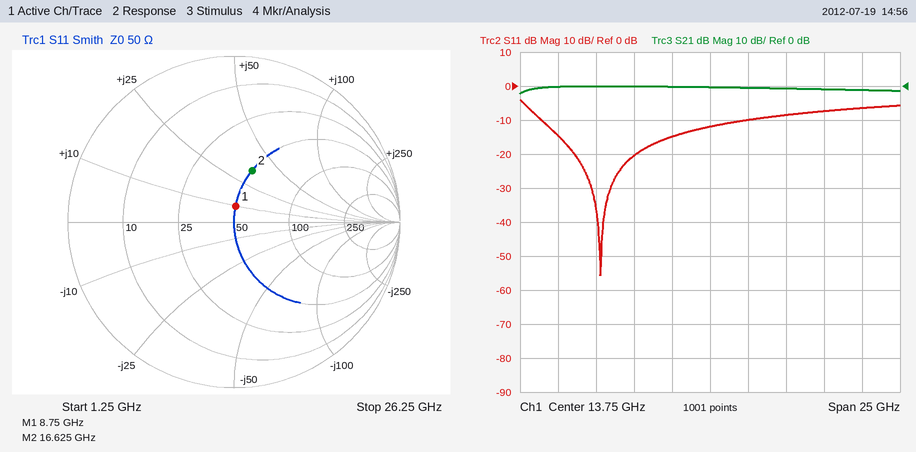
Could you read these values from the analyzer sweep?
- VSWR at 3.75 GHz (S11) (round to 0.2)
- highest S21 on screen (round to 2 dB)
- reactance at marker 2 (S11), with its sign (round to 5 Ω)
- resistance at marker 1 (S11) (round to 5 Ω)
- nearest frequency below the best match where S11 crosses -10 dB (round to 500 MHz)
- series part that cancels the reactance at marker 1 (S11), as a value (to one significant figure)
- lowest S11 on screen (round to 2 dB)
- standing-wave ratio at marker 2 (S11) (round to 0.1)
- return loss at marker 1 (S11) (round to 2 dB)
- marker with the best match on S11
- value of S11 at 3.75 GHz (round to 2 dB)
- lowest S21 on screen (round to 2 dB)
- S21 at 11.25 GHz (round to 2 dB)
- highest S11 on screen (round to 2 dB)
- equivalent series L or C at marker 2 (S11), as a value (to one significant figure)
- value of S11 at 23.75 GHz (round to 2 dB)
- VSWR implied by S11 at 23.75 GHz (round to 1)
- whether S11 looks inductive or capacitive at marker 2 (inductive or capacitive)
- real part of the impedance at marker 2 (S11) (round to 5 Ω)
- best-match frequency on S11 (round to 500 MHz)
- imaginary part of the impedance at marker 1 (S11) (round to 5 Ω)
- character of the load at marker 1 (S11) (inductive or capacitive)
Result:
1.4
0 dB
+35 Ω
50 Ω
2.5 GHz
2 pF
-56 dB
2.0
20 dB
marker 1
-14 dB
-2 dB
0 dB
-4 dB
300 pH
-6 dB
3
inductive
50 Ω
6.5 GHz
+10 Ω
inductive
